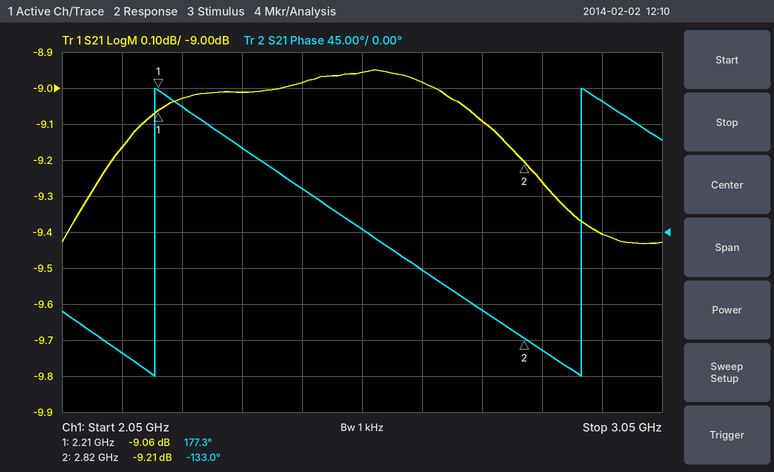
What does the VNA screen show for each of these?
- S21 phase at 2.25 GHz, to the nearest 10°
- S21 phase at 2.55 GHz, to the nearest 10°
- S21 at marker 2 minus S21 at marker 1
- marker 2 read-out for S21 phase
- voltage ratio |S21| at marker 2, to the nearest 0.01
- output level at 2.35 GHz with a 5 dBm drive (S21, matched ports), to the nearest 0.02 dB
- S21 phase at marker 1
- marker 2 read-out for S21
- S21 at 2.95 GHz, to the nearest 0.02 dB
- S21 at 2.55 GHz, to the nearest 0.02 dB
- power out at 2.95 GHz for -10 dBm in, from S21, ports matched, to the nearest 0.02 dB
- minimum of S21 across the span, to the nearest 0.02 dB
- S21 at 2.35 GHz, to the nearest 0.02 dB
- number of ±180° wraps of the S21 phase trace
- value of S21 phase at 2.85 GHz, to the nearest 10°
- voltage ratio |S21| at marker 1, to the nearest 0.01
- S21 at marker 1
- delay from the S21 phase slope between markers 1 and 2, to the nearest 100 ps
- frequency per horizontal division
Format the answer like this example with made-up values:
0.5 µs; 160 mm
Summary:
160°; 0°; -0.15 dB; -133.0°; 0.35; -4.02 dBm; 177.3°; -9.21 dB; -9.40 dB; -8.96 dB; -19.40 dBm; -9.44 dB; -9.02 dB; 2; -150°; 0.35; -9.06 dB; 1.4 ns; 100 MHz
